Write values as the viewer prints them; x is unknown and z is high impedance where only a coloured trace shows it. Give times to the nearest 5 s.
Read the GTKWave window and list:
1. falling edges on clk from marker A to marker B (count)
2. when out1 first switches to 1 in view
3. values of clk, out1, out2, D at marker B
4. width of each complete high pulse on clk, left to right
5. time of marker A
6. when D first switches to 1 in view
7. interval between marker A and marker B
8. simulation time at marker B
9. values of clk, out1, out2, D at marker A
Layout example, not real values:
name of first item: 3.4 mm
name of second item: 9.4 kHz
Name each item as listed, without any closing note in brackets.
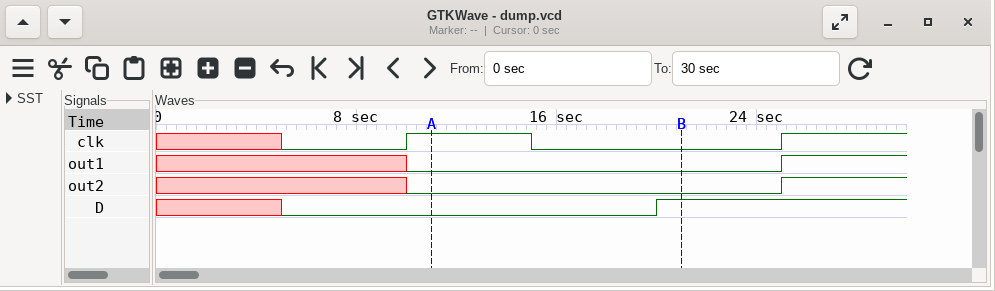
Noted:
falling edges on clk from marker A to marker B: 1
when out1 first switches to 1 in view: 25 s
values of clk, out1, out2, D at marker B: clk=0, out1=0, out2=0, D=1
width of each complete high pulse on clk, left to right: 5 s
time of marker A: 10 s
when D first switches to 1 in view: 20 s
interval between marker A and marker B: 10 s
simulation time at marker B: 20 s
values of clk, out1, out2, D at marker A: clk=1, out1=0, out2=0, D=0
